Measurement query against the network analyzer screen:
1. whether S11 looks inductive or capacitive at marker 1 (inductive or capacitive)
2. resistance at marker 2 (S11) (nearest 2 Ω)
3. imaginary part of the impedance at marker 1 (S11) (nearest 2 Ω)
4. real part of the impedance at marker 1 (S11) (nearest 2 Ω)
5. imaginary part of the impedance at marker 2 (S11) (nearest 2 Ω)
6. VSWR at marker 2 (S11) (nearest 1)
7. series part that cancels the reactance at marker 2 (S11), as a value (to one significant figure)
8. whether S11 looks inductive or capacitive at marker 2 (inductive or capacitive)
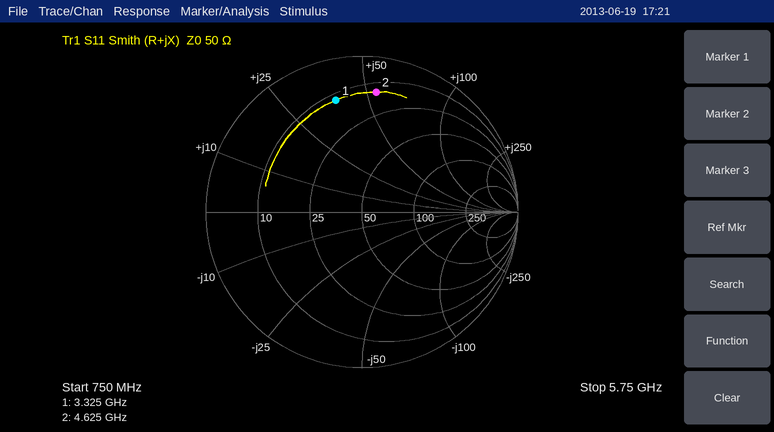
inductive
14 Ω
+38 Ω
12 Ω
+54 Ω
8
600 fF
inductive
